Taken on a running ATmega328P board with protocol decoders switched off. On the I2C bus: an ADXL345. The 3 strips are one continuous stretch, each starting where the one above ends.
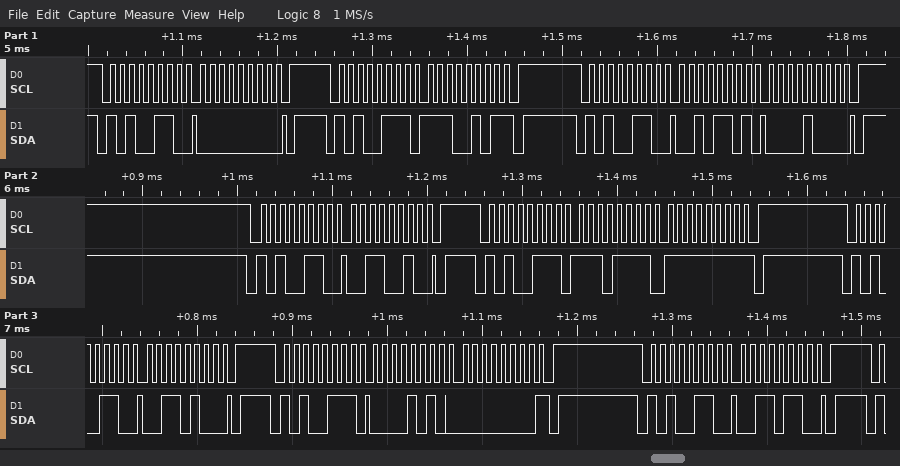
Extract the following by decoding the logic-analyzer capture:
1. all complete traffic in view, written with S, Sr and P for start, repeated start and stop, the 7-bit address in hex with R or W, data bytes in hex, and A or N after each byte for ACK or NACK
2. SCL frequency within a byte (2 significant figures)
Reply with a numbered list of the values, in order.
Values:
1. S 53W A 00 A P S 53R A E5 N P S 53W A 2D A 08 A P S 53W A 32 A P S 53R A EF A FF N P S 53W A 34 A P S 53R A 0A A 00 N P S 53W A 36 A P
2. 100 kHz
